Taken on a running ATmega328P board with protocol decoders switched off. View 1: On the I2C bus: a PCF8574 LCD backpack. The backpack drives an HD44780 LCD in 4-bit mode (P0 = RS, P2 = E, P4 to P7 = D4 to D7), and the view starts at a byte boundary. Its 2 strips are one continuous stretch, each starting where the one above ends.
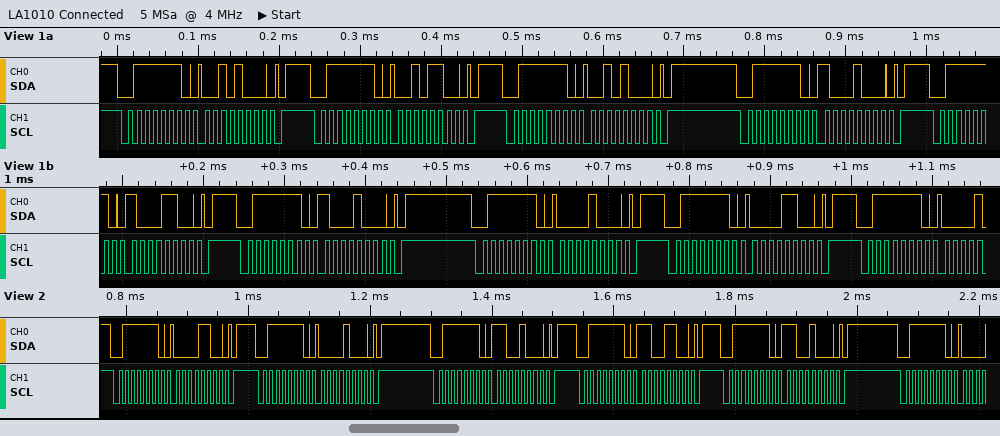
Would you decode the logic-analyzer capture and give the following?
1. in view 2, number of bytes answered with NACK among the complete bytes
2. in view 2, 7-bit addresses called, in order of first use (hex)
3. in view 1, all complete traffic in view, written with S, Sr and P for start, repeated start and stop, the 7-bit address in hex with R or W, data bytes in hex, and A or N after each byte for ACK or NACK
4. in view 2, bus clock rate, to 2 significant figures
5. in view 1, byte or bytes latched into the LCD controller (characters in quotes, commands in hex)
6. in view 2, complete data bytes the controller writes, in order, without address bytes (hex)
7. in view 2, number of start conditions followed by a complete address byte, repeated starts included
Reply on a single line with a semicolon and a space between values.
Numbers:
0; 0x3F; S 3FW A 28 A P S 3FW A 2C A P S 3FW A 28 A P S 3FW A 88 A P S 3FW A 8C A P S 3FW A 88 A P S 3FW A 08 A P S 3FW A 0C A P S 3FW A; 100 kHz; 0x28; 0C 08 C8 CC C8; 6
